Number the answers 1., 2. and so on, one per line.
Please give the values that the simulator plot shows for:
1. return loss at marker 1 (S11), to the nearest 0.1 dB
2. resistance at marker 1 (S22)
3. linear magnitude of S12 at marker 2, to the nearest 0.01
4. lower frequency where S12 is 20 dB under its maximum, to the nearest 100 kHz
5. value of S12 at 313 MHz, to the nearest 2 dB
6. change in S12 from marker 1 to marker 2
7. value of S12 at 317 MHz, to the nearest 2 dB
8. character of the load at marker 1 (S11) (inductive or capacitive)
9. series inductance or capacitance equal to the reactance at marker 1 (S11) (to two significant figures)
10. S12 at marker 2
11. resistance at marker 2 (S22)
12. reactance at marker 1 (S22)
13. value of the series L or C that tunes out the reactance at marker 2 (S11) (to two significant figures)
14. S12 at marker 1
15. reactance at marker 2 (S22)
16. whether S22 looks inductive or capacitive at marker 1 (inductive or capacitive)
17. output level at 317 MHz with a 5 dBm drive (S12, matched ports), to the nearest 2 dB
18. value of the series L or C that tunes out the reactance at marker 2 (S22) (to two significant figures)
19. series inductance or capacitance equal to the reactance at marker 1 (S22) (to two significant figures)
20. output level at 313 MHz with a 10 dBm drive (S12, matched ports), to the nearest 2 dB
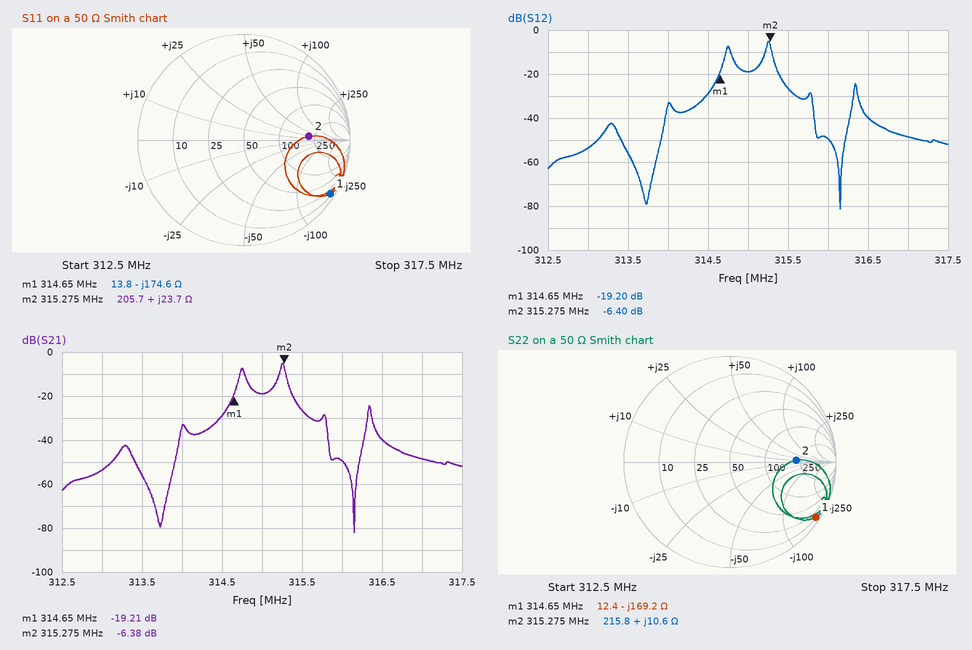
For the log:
1. 0.4 dB
2. 12.4 Ω
3. 0.48
4. 314.6 MHz
5. -54 dB
6. 12.80 dB
7. -48 dB
8. capacitive
9. 2.9 pF
10. -6.40 dB
11. 215.8 Ω
12. -169.2 Ω
13. 21 pF
14. -19.20 dB
15. +10.6 Ω
16. capacitive
17. -44 dBm
18. 48 pF
19. 3.0 pF
20. -44 dBm
